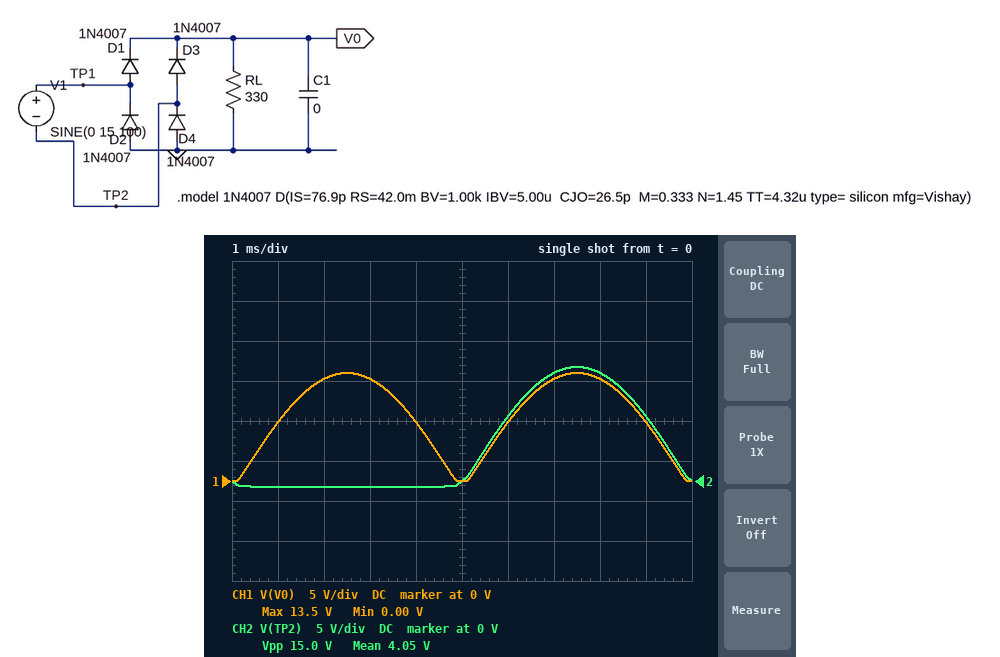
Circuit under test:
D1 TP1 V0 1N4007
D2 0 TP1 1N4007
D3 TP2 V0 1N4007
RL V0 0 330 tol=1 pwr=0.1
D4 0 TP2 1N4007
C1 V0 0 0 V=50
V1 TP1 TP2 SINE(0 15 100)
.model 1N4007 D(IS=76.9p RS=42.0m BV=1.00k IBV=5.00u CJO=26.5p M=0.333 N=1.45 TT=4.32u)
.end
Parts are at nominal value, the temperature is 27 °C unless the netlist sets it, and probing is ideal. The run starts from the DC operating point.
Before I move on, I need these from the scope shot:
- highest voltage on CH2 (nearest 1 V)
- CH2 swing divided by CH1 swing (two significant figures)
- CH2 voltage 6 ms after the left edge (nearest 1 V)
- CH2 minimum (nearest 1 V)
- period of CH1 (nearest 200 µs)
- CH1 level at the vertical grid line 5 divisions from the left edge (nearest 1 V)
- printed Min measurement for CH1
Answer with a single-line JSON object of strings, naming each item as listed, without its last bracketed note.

{"highest voltage on CH2": "14 V", "CH2 swing divided by CH1 swing": "1.1", "CH2 voltage 6 ms after the left edge": "8 V", "CH2 minimum": "-1 V", "period of CH1": "5.0 ms", "CH1 level at the vertical grid line 5 divisions from the left edge": "0 V", "printed Min measurement for CH1": "0.00 V"}
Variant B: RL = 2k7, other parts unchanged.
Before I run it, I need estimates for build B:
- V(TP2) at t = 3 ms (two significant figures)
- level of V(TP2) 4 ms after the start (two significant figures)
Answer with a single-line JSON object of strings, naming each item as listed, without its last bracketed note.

{"V(TP2) at t = 3 ms": "-670 mV", "level of V(TP2) 4 ms after the start": "-650 mV"}
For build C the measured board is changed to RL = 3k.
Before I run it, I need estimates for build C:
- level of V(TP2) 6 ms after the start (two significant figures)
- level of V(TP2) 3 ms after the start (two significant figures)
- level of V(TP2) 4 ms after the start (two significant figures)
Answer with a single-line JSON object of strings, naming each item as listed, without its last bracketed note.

{"level of V(TP2) 6 ms after the start": "8.2 V", "level of V(TP2) 3 ms after the start": "-670 mV", "level of V(TP2) 4 ms after the start": "-650 mV"}
